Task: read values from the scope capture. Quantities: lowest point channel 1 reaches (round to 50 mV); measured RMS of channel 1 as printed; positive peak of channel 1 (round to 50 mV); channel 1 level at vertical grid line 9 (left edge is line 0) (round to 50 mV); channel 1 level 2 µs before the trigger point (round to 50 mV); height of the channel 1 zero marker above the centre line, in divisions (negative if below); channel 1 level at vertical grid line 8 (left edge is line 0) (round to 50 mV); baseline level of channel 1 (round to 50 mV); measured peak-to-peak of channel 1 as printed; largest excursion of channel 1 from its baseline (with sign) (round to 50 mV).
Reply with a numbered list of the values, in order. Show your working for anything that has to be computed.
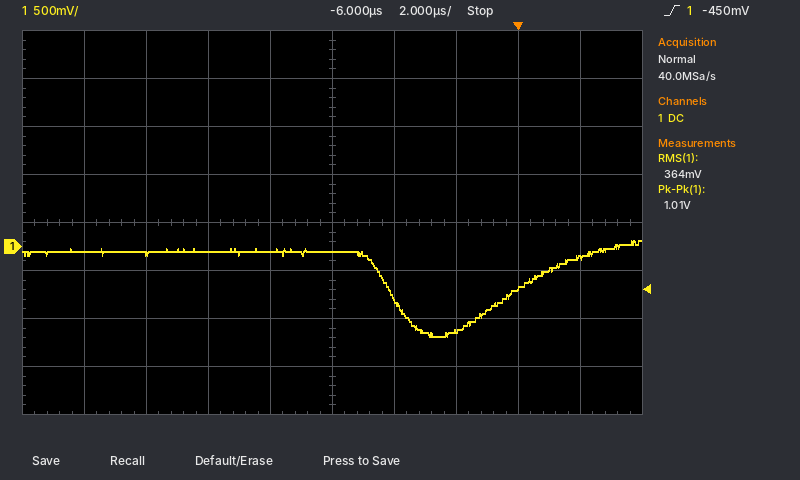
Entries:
1. -950 mV
2. 364 mV
3. 50 mV
4. -100 mV
5. -900 mV
6. -0.5 div
7. -450 mV
8. -50 mV
9. 1.01 V
10. -950 mV − (-50 mV) = -900 mV
